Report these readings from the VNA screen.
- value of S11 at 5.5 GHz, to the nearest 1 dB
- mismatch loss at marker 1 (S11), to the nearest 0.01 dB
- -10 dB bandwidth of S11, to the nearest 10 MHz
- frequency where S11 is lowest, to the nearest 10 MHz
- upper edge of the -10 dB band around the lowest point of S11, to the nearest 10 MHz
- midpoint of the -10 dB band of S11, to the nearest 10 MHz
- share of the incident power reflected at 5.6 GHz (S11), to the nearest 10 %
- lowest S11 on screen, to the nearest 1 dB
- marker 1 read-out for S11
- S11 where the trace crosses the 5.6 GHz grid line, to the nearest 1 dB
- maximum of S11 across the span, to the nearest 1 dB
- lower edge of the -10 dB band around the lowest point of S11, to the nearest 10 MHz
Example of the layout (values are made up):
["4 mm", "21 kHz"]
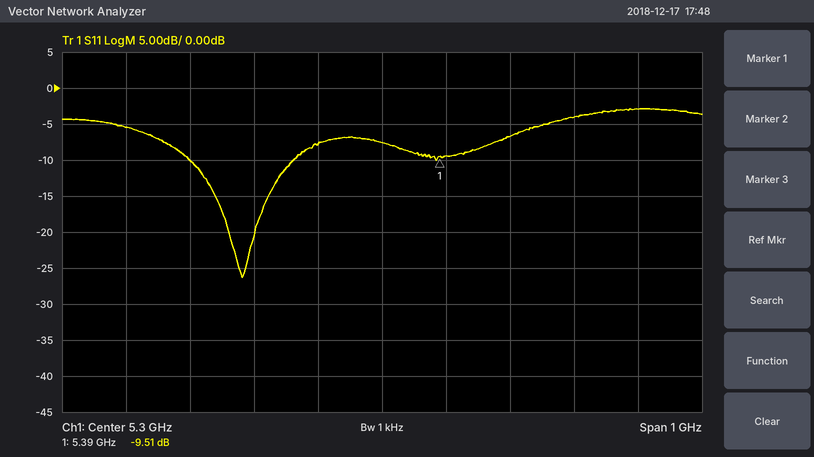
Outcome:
["-7 dB", "0.52 dB", "160 MHz", "5.08 GHz", "5.16 GHz", "5.08 GHz", "40 %", "-26 dB", "-9.51 dB", "-4 dB", "-3 dB", "5.00 GHz"]
